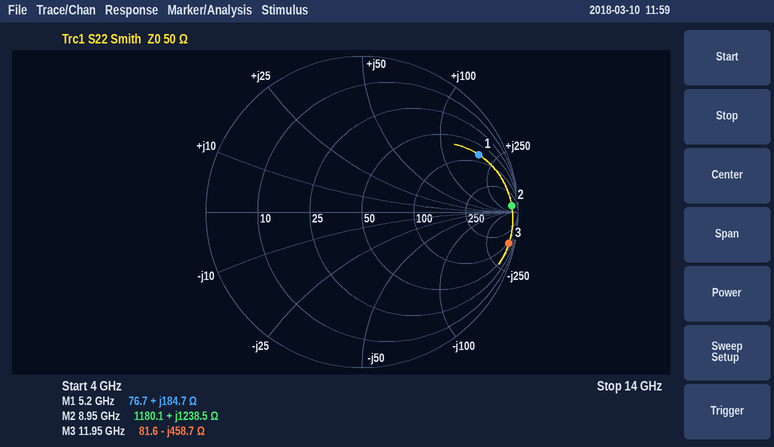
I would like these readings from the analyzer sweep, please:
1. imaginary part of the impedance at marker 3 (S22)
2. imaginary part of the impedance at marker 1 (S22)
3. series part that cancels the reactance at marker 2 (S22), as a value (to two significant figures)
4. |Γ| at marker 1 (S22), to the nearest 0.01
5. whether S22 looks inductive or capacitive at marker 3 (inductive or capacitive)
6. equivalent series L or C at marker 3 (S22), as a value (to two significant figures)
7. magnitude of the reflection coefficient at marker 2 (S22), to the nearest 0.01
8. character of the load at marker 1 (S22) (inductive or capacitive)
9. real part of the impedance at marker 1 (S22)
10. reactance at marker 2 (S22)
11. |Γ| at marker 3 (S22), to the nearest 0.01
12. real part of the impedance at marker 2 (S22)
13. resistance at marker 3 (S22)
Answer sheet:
-458.7 Ω
+184.7 Ω
14 fF
0.83
capacitive
29 fF
0.96
inductive
76.7 Ω
+1238.5 Ω
0.96
1180.1 Ω
81.6 Ω
